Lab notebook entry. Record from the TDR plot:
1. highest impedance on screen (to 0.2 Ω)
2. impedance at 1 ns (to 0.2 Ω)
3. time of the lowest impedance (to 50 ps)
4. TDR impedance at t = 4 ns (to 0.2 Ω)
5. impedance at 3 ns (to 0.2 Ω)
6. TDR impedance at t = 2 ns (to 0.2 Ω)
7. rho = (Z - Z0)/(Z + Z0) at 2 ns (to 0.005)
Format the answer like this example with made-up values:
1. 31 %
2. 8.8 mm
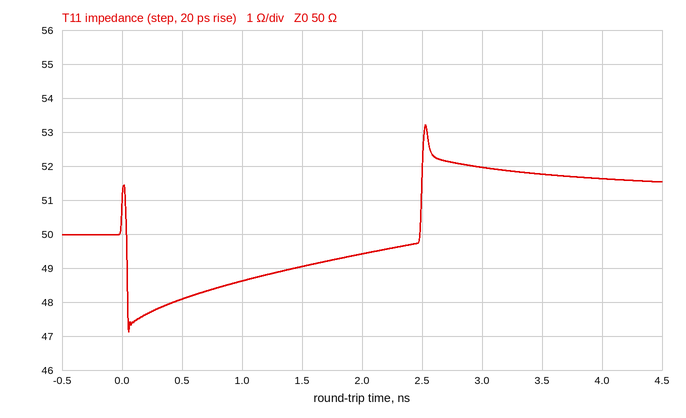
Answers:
1. 53.2 Ω
2. 48.6 Ω
3. 50 ps
4. 51.6 Ω
5. 52.0 Ω
6. 49.4 Ω
7. -0.005
